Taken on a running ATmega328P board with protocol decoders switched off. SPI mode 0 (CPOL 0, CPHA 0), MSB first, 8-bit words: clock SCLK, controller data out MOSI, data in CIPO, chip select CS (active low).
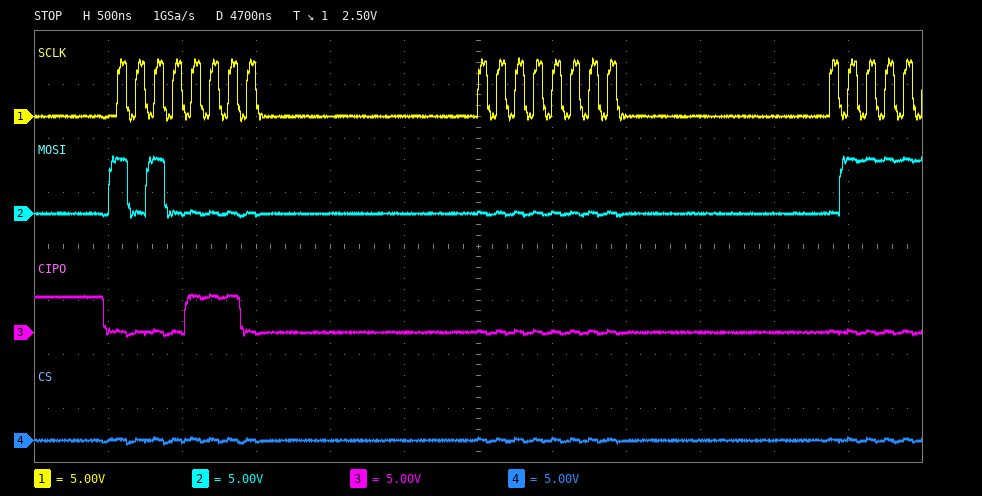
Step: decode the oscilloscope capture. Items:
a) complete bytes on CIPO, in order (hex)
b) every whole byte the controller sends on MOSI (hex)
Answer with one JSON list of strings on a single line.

["0E 00", "A0 00"]
